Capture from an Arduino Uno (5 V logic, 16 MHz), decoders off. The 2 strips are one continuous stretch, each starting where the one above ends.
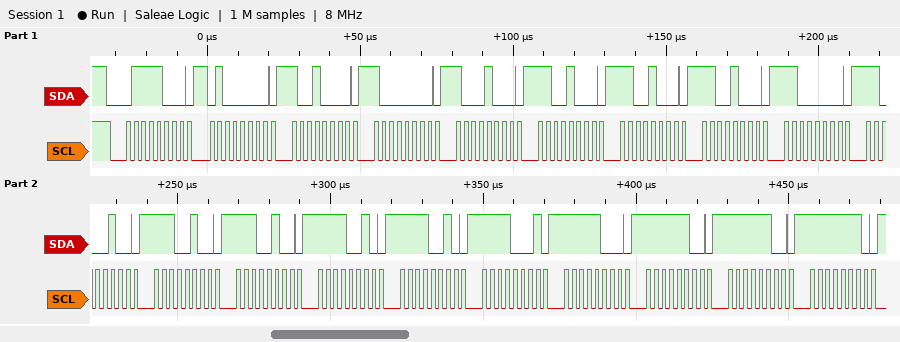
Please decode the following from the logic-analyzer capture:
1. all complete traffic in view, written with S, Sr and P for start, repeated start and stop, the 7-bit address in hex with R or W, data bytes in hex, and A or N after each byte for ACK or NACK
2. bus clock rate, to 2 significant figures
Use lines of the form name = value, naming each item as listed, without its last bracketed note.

all complete traffic in view, written with S, Sr and P for start, repeated start and stop, the 7-bit address in hex with R or W, data bytes in hex, and A or N after each byte for ACK or NACK = S 3CW A 40 A 90 A 80 A 88 A C8 A C8 A C8 A C0 A C4 A E4 A E4 A F2 A F2 A F1 A F8 A FC A FC A FE A
bus clock rate, to 2 significant figures = 400 kHz
